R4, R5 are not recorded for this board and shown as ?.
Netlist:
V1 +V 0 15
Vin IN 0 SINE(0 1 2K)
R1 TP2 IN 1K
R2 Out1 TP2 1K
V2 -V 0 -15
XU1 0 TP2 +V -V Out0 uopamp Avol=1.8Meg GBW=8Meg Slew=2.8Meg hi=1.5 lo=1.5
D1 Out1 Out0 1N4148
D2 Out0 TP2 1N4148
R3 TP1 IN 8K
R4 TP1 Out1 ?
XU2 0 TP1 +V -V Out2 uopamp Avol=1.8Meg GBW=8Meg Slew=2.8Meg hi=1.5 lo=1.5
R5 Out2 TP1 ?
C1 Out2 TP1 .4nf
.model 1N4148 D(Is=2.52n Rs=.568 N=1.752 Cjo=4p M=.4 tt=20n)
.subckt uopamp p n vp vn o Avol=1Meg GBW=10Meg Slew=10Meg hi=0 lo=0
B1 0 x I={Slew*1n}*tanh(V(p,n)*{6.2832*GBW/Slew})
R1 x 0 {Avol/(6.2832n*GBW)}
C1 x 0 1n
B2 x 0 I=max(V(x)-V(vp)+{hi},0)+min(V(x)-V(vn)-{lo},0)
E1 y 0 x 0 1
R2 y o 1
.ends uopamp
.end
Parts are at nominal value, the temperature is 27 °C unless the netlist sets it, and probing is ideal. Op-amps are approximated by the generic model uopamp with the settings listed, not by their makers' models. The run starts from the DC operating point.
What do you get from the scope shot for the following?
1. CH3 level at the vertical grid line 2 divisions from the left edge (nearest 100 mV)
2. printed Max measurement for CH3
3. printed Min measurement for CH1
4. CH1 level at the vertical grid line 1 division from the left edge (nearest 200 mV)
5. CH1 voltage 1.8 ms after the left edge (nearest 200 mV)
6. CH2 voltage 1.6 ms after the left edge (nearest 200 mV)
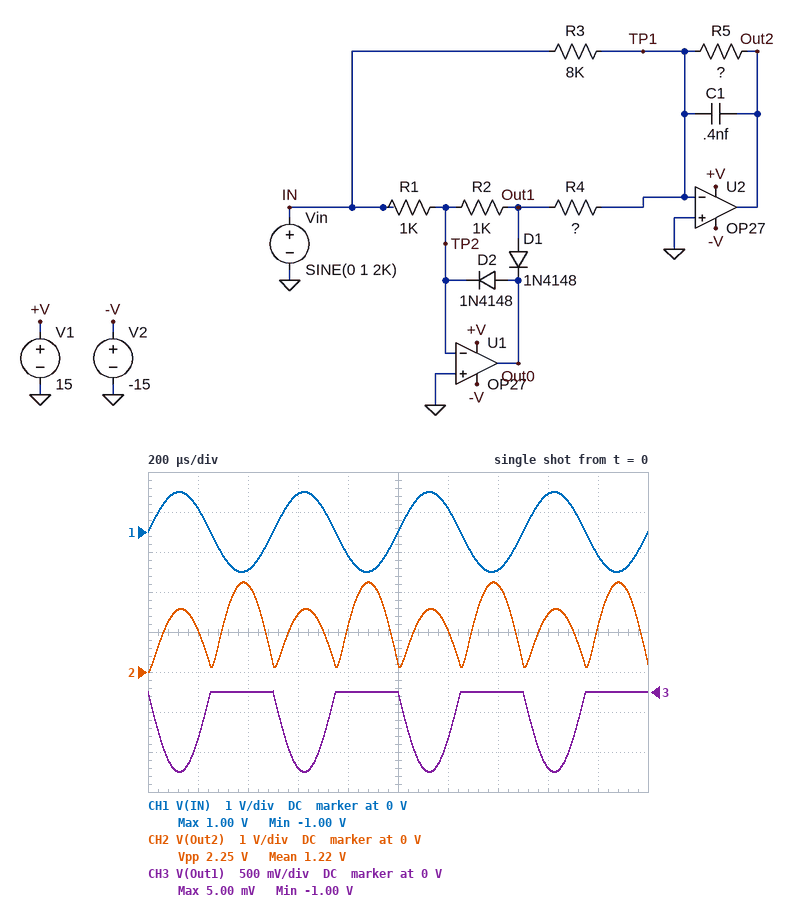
0 V
5.00 mV
-1.00 V
600 mV
-600 mV
1.4 V
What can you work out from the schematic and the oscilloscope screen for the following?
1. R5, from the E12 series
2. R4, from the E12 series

18 kΩ
4.7 kΩ
